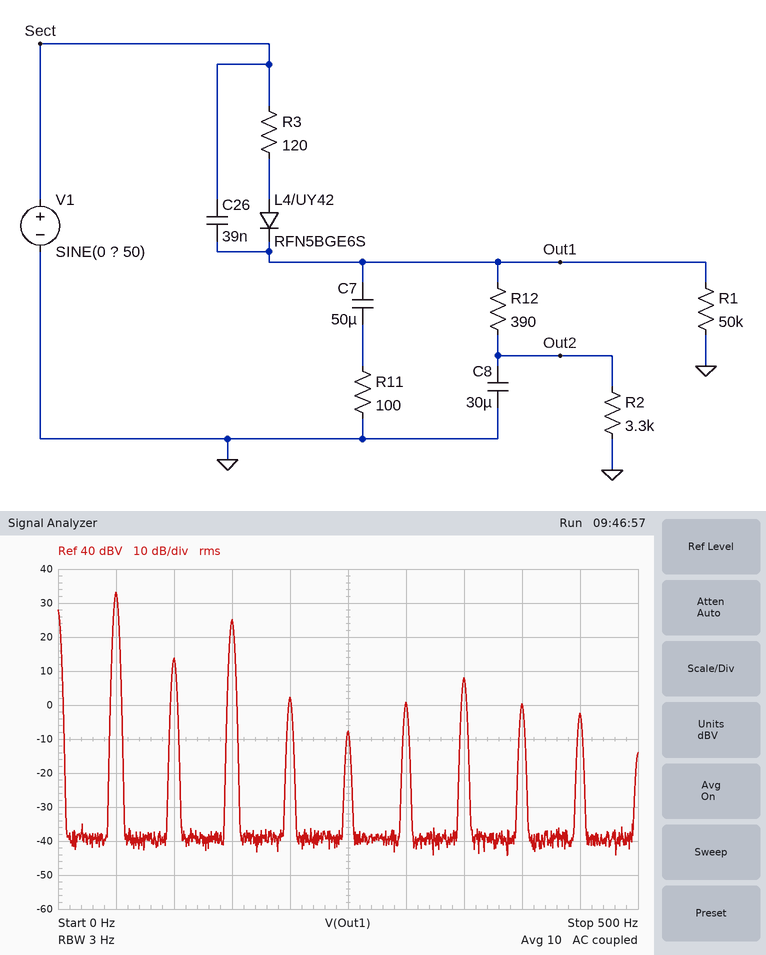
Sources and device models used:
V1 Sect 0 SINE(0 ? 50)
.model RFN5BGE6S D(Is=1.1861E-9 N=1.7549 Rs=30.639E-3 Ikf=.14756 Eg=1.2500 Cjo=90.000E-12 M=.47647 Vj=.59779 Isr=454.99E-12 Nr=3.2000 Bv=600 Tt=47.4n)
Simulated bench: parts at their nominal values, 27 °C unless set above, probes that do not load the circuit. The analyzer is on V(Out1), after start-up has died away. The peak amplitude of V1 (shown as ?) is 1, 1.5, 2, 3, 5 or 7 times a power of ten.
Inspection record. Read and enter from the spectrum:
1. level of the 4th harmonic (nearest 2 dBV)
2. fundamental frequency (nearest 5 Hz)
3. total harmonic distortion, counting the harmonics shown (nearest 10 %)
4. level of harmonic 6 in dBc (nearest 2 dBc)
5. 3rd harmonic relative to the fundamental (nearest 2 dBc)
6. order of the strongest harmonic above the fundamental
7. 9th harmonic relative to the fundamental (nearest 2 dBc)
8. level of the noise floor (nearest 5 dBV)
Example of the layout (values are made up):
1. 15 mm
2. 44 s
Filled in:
1. 2 dBV
2. 50 Hz
3. 40 %
4. -32 dBc
5. -8 dBc
6. 3
7. -36 dBc
8. -40 dBV
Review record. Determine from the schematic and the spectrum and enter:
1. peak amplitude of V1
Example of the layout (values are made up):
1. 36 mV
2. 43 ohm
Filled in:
1. 500 V
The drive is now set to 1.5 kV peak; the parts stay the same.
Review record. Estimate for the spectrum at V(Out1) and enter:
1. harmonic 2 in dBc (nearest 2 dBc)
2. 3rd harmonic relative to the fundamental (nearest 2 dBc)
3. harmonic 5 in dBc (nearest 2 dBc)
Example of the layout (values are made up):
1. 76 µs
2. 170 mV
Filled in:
1. -48 dBc
2. -20 dBc
3. -26 dBc
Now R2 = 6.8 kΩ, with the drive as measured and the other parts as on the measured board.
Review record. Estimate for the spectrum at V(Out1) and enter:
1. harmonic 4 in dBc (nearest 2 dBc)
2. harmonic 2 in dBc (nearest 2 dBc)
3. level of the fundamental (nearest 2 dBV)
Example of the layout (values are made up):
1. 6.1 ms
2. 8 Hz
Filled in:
1. -36 dBc
2. -24 dBc
3. 34 dBV
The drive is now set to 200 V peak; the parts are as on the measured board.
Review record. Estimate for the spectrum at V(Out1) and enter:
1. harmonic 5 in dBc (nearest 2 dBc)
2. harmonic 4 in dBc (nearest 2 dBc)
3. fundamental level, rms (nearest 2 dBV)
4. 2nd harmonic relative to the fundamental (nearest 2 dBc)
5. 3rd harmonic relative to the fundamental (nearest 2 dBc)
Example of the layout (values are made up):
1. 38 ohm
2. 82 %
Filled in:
1. -18 dBc
2. -10 dBc
3. 14 dBV
4. -2 dBc
5. -6 dBc
